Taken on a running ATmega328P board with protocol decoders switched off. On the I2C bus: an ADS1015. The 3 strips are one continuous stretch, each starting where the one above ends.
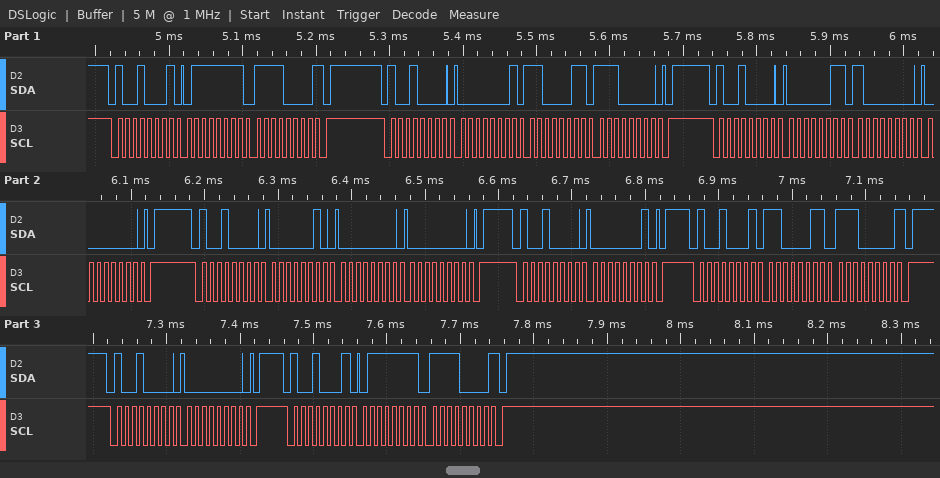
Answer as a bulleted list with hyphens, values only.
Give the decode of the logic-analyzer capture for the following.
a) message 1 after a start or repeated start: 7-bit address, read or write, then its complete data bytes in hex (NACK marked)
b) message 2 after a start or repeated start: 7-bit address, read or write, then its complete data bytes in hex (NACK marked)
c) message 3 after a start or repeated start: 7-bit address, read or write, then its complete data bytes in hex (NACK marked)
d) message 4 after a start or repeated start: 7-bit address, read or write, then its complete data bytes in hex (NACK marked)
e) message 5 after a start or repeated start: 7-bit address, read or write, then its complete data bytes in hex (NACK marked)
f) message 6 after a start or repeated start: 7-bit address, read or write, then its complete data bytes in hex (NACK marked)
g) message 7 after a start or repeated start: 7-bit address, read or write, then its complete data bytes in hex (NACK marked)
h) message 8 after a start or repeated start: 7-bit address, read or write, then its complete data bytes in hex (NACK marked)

- 0x48 read: 7F F0 NACK
- 0x48 write: 01 C3 E0
- 0x48 write: 03 80 00
- 0x48 write: 02 00 00
- 0x48 write: 01
- 0x48 read: C3 E0 NACK
- 0x48 write: 00
- 0x48 read: 7F F0 NACK
